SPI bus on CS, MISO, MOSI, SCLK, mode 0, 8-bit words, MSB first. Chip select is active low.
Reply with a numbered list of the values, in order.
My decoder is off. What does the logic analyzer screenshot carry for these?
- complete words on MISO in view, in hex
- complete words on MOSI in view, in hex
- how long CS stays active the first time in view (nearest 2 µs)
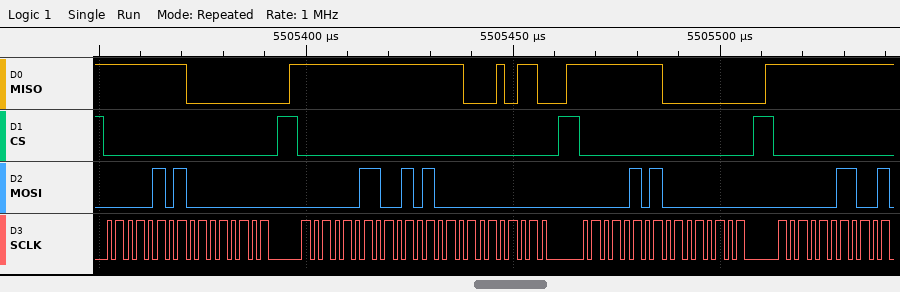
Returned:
1. FF, 00, FF, FF, 16, FF, 00, FF
2. 05, 00, 03, 28, 00, 05, 00, 03
3. 42 µs
